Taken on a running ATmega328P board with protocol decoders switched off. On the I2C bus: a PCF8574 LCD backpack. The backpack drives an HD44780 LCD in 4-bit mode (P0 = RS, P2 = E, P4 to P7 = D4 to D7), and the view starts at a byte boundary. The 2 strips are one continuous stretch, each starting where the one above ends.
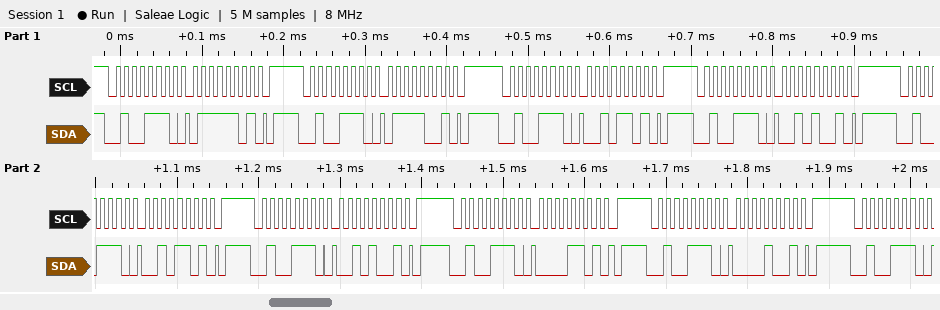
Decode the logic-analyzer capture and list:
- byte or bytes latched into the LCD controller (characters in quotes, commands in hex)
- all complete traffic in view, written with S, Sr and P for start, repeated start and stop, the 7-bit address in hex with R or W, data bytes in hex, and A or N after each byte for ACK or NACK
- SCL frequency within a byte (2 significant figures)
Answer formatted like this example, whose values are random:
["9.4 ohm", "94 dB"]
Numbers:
["'r' ' '", "S 27W A 7D A P S 27W A 79 A P S 27W A 2D A P S 27W A 29 A P S 27W A 2D A P S 27W A 29 A P S 27W A 0D A P S 27W A 09 A P S 27W A", "100 kHz"]
